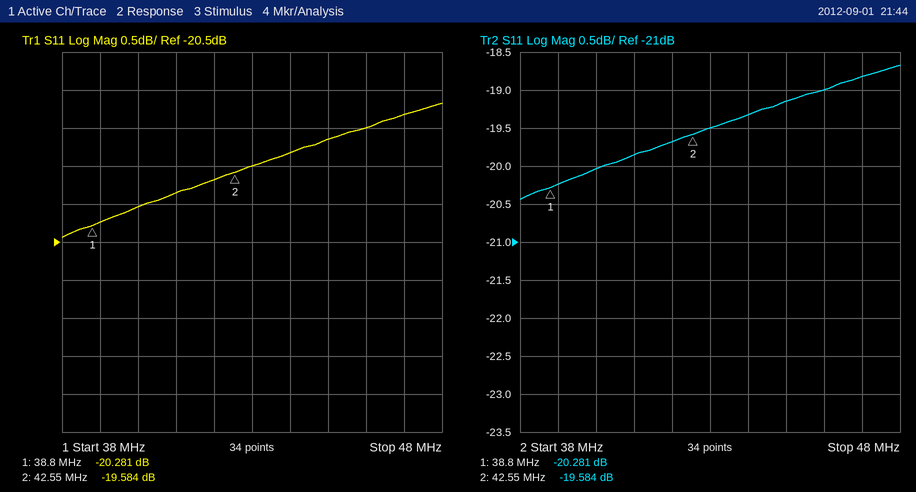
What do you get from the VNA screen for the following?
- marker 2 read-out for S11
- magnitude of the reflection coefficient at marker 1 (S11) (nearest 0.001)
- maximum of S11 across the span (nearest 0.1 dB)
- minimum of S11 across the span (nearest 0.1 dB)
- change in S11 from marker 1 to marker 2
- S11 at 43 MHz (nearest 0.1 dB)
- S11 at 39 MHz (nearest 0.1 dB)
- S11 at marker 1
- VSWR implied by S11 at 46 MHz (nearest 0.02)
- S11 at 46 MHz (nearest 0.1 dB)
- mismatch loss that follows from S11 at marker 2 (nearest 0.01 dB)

-19.584 dB
0.097
-18.7 dB
-20.4 dB
0.697 dB
-19.5 dB
-20.2 dB
-20.281 dB
1.26
-19.0 dB
0.05 dB
